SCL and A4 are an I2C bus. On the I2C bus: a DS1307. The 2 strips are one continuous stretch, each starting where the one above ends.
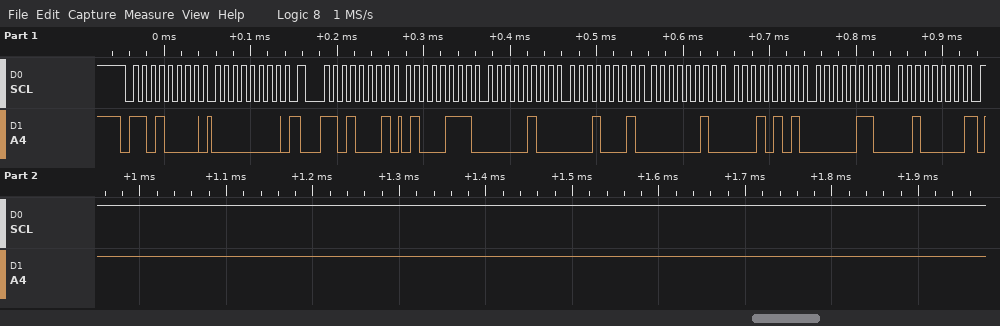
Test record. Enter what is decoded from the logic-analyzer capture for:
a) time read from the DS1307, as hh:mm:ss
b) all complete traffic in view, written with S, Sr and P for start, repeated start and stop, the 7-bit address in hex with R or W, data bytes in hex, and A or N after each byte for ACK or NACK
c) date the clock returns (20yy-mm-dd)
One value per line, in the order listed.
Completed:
11:04:47
S 68W A 00 A Sr 68R A 47 A 04 A 11 A 02 A 15 A 06 A 20 N P
2020-06-15
